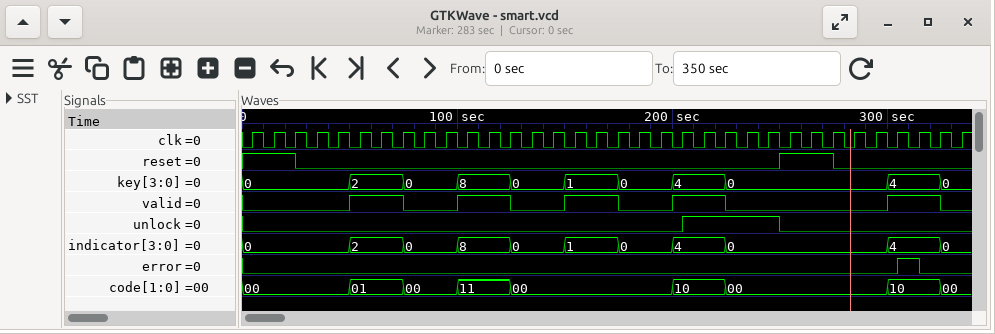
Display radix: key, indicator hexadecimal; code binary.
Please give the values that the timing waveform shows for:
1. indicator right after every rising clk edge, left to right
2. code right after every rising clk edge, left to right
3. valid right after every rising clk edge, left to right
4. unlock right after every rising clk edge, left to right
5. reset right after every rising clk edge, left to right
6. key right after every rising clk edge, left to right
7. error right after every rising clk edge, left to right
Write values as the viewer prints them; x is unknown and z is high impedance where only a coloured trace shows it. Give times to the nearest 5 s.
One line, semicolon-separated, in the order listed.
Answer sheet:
0, 0, 0, 0, 0, 2, 2, 0, 0, 0, 8, 8, 0, 0, 0, 1, 1, 0, 0, 0, 4, 4, 0, 0, 0, 0, 0, 0, 0, 0, 4, 4, 0, 0; 00, 00, 00, 00, 00, 01, 01, 00, 00, 00, 11, 11, 00, 00, 00, 00, 00, 00, 00, 00, 10, 10, 00, 00, 00, 00, 00, 00, 00, 00, 10, 10, 00, 00; 0 0 0 0 0 1 1 0 0 0 1 1 0 0 0 1 1 0 0 0 1 1 0 0 0 0 0 0 0 0 1 1 0 0; 0 0 0 0 0 0 0 0 0 0 0 0 0 0 0 0 0 0 0 0 1 1 1 1 1 0 0 0 0 0 0 0 0 0; 1 1 0 0 0 0 0 0 0 0 0 0 0 0 0 0 0 0 0 0 0 0 0 0 0 1 1 0 0 0 0 0 0 0; 0, 0, 0, 0, 0, 2, 2, 0, 0, 0, 8, 8, 0, 0, 0, 1, 1, 0, 0, 0, 4, 4, 0, 0, 0, 0, 0, 0, 0, 0, 4, 4, 0, 0; 0 0 0 0 0 0 0 0 0 0 0 0 0 0 0 0 0 0 0 0 0 0 0 0 0 0 0 0 0 0 1 0 0 0
